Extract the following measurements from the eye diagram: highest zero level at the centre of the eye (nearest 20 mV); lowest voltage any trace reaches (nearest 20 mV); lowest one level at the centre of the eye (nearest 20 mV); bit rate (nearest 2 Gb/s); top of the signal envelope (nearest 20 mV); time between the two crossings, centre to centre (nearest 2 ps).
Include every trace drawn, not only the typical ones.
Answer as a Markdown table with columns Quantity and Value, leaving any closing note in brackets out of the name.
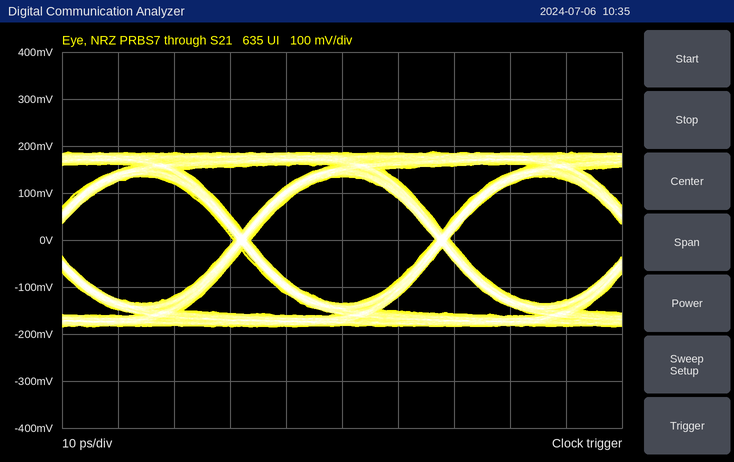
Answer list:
| Quantity | Value |
|---|---|
| highest zero level at the centre of the eye | -140 mV |
| lowest voltage any trace reaches | -180 mV |
| lowest one level at the centre of the eye | 140 mV |
| bit rate | 28 Gb/s |
| top of the signal envelope | 180 mV |
| time between the two crossings, centre to centre | 36 ps |
